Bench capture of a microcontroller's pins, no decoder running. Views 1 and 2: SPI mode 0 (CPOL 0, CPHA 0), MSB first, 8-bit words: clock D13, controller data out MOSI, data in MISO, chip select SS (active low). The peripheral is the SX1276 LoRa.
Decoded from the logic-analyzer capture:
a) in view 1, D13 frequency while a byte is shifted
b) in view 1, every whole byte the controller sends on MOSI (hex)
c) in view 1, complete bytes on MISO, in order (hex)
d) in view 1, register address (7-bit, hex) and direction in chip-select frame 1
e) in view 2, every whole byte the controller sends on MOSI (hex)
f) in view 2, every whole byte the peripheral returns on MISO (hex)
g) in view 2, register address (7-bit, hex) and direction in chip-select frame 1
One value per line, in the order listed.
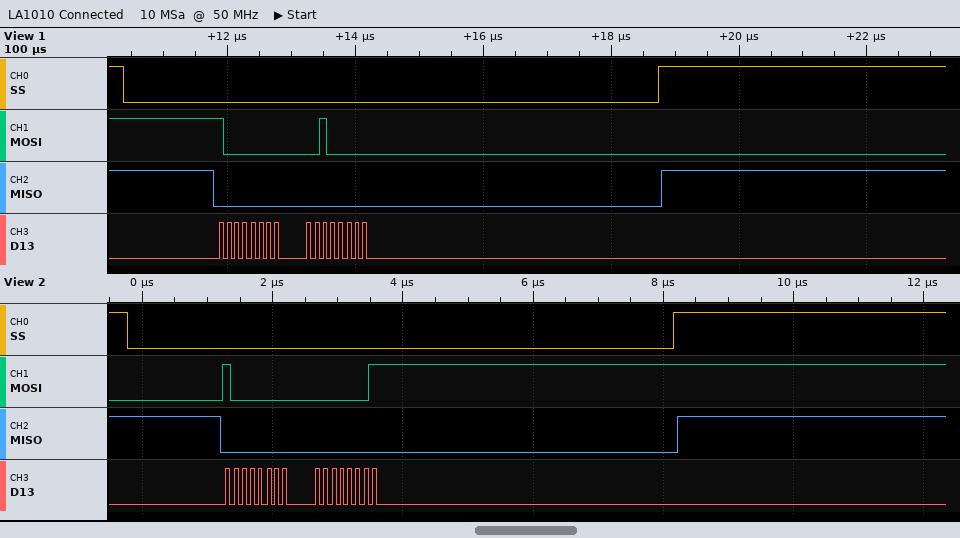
8 MHz
0x80 0x20
0x00 0x00
0x00 write
80 01
00 00
0x00 write
